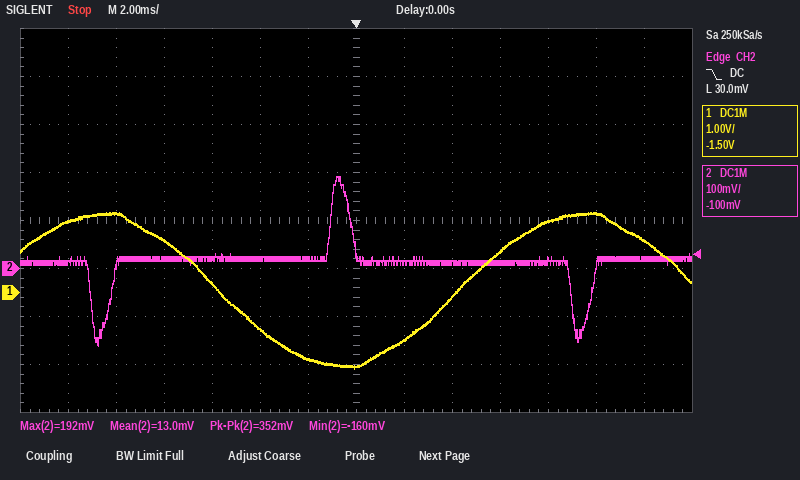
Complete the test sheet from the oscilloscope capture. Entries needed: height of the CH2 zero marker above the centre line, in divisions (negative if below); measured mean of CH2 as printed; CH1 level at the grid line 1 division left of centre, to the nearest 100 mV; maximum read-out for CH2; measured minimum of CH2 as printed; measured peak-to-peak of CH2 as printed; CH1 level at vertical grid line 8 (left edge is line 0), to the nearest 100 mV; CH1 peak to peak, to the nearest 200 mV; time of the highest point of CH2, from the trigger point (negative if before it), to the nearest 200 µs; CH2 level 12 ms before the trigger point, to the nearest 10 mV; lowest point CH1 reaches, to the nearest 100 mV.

-1.0 div
13.0 mV
-1.4 V
192 mV
-160 mV
352 mV
-1.0 V
3.2 V
-800 µs
10 mV
-1.6 V
